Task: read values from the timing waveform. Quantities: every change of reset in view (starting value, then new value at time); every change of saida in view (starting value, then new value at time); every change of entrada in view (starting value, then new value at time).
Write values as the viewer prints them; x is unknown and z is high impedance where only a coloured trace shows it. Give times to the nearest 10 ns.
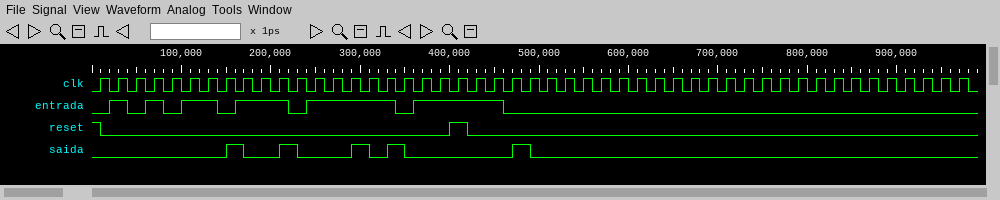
1, 0 at 10 ns, 1 at 400 ns, 0 at 420 ns
0, 1 at 150 ns, 0 at 170 ns, 1 at 210 ns, 0 at 230 ns, 1 at 290 ns, 0 at 310 ns, 1 at 330 ns, 0 at 350 ns, 1 at 470 ns, 0 at 490 ns
0, 1 at 20 ns, 0 at 40 ns, 1 at 60 ns, 0 at 80 ns, 1 at 100 ns, 0 at 140 ns, 1 at 160 ns, 0 at 220 ns, 1 at 240 ns, 0 at 340 ns, 1 at 360 ns, 0 at 460 ns
